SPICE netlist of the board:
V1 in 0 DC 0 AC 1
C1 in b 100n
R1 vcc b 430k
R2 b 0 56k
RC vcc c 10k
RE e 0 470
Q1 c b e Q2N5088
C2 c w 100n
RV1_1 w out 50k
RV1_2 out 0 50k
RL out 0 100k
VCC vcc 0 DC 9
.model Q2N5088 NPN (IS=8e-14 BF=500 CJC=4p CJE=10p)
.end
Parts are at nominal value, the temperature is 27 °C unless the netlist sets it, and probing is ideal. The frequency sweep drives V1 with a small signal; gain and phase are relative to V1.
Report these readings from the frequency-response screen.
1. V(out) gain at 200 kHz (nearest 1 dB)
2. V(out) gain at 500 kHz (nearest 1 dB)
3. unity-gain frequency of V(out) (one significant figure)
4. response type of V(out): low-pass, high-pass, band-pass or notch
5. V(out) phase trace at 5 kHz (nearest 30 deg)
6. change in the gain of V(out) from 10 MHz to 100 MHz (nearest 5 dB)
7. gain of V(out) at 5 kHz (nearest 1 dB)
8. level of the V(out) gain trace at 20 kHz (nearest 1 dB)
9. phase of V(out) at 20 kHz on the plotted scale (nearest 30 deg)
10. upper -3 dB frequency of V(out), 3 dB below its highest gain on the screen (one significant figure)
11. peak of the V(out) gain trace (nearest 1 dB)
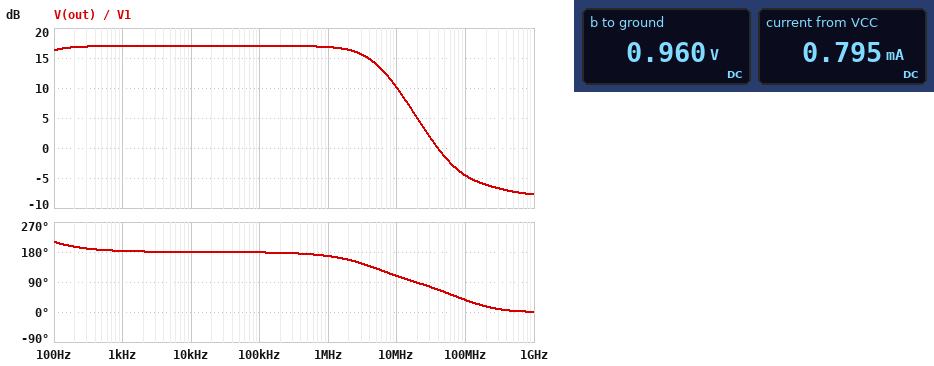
17 dB
17 dB
40 MHz
low-pass
180 deg
-15 dB
17 dB
17 dB
180 deg
5 MHz
17 dB
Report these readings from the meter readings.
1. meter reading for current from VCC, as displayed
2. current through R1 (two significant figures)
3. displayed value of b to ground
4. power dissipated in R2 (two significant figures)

0.795 mA
19 µA
0.960 V
16 µW
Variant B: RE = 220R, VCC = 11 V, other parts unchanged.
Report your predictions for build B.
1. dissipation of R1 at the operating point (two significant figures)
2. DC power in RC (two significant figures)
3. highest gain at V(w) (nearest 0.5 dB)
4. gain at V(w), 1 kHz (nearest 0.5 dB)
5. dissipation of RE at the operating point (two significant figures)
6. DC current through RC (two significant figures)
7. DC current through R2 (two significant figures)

240 µW
11 mW
20.0 dB
7.0 dB
250 µW
1.1 mA
15 µA
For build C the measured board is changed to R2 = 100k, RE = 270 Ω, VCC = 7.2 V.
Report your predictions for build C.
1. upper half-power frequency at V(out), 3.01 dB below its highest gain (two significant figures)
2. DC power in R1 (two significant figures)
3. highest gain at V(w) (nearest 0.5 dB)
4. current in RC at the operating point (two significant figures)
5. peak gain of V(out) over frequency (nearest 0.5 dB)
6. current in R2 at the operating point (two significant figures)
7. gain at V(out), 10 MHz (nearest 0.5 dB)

11 MHz
96 µW
18.5 dB
690 µA
10.5 dB
7.8 µA
7.5 dB
